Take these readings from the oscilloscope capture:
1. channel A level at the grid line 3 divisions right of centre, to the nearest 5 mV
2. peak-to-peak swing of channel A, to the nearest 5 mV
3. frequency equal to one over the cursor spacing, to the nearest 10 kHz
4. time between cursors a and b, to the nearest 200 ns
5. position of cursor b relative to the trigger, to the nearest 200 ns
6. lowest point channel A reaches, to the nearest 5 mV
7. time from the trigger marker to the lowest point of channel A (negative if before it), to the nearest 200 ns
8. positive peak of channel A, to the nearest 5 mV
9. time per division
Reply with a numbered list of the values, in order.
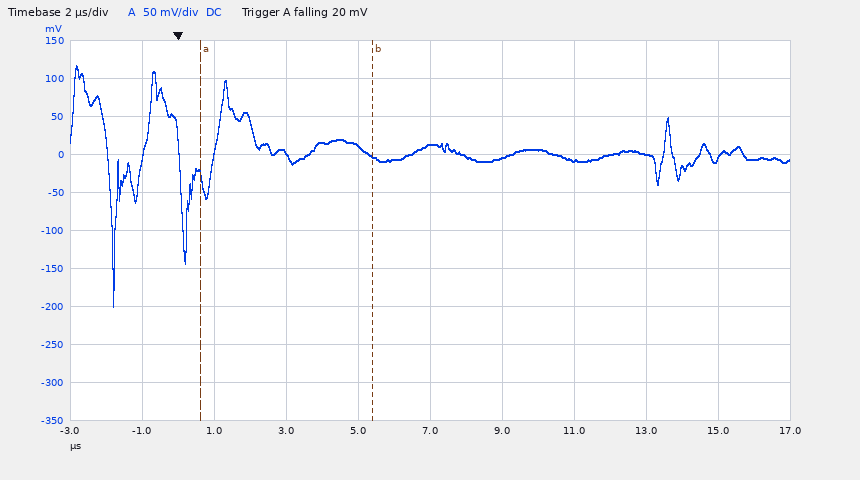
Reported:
1. 0 mV
2. 315 mV
3. 210 kHz
4. 4.8 µs
5. +5.4 µs
6. -200 mV
7. -1.8 µs
8. 115 mV
9. 2 µs
